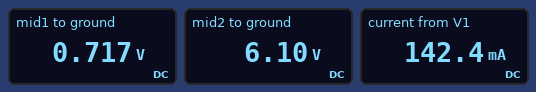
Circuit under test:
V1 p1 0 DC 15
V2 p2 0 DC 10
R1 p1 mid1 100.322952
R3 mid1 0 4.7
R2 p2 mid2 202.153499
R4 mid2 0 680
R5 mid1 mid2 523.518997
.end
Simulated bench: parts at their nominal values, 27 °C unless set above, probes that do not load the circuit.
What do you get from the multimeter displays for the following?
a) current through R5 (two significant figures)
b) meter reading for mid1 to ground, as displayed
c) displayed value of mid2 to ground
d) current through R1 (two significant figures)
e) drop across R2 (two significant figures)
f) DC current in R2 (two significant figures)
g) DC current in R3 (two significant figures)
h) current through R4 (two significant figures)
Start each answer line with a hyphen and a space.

- 10 mA
- 0.717 V
- 6.10 V
- 140 mA
- 3.9 V
- 19 mA
- 150 mA
- 9.0 mA
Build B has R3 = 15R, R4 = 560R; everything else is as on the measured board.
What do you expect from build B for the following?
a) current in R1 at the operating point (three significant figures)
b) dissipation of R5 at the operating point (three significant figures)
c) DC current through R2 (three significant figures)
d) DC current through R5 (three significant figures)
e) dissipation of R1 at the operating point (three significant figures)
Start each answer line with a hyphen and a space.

- 129 mA
- 32.5 mW
- 18.9 mA
- 7.88 mA
- 1.67 W
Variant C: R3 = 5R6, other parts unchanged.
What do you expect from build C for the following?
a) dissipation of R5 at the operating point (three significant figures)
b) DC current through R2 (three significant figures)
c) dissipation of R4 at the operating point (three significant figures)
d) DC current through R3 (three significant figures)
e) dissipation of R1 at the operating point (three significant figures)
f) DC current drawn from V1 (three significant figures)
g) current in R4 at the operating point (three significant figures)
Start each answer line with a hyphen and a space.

- 53.4 mW
- 19.1 mA
- 55.3 mW
- 151 mA
- 2.00 W
- 141 mA
- 9.02 mA
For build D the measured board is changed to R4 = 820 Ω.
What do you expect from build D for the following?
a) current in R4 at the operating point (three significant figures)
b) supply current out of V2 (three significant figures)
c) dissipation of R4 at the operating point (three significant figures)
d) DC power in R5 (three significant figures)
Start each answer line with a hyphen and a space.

- 7.68 mA
- 18.3 mA
- 48.3 mW
- 59.4 mW
